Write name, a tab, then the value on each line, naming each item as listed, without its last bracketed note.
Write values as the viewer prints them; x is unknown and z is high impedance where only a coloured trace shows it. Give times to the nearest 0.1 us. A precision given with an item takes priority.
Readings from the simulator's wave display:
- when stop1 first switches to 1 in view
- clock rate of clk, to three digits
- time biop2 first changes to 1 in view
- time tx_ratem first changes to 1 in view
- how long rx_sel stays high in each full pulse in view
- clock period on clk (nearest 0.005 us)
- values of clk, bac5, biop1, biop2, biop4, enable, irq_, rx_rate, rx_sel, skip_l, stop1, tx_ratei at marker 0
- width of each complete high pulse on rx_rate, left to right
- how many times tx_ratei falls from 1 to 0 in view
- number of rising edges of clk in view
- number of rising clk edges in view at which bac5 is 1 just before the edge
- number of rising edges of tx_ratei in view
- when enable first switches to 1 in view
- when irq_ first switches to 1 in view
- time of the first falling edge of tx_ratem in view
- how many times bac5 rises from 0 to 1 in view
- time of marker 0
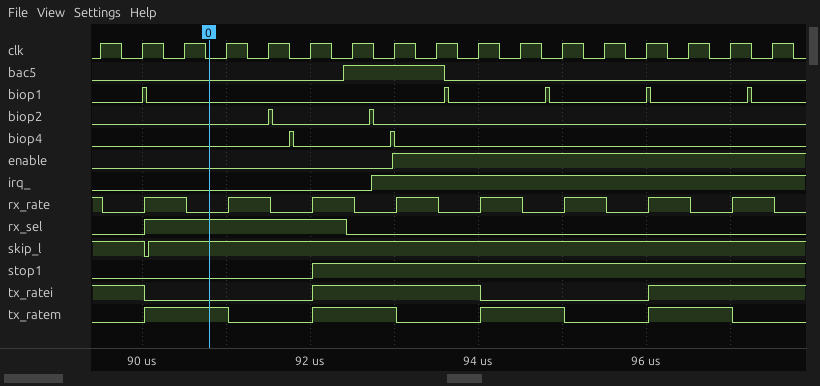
when stop1 first switches to 1 in view	92 us
clock rate of clk, to three digits	2.00 MHz
time biop2 first changes to 1 in view	91.5 us
time tx_ratem first changes to 1 in view	90 us
how long rx_sel stays high in each full pulse in view	2.4 us
clock period on clk	0.5 us
values of clk, bac5, biop1, biop2, biop4, enable, irq_, rx_rate, rx_sel, skip_l, stop1, tx_ratei at marker 0	clk=0, bac5=0, biop1=0, biop2=0, biop4=0, enable=0, irq_=0, rx_rate=0, rx_sel=1, skip_l=1, stop1=0, tx_ratei=0
width of each complete high pulse on rx_rate, left to right	0.5 us, 0.5 us, 0.5 us, 0.5 us, 0.5 us, 0.5 us, 0.5 us, 0.5 us
how many times tx_ratei falls from 1 to 0 in view	2
number of rising edges of clk in view	17
number of rising clk edges in view at which bac5 is 1 just before the edge	3
number of rising edges of tx_ratei in view	2
when enable first switches to 1 in view	93 us
when irq_ first switches to 1 in view	92.7 us
time of the first falling edge of tx_ratem in view	91 us
how many times bac5 rises from 0 to 1 in view	1
time of marker 0	90.8 us
